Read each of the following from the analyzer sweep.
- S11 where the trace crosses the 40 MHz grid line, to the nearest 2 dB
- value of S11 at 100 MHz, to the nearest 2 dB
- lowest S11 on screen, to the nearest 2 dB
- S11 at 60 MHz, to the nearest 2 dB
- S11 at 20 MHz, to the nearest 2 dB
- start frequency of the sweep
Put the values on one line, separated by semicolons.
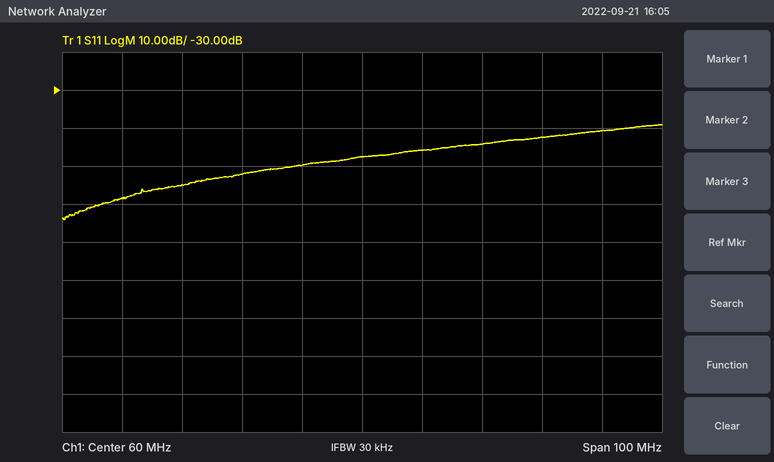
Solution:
-52 dB; -40 dB; -64 dB; -48 dB; -58 dB; 10 MHz
